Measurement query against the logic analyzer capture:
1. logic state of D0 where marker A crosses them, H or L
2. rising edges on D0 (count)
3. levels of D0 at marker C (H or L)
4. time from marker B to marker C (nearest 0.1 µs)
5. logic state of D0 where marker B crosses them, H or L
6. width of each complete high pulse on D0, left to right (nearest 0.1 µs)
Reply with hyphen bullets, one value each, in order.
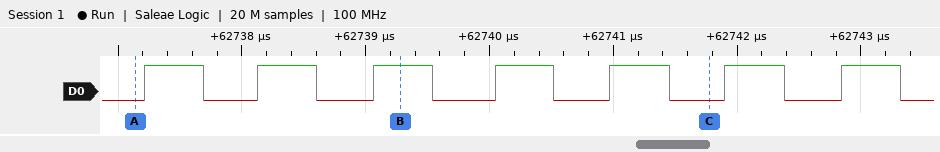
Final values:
- D0=L
- 7
- D0=L
- 2.5 µs
- D0=H
- 0.5 µs, 0.5 µs, 0.5 µs, 0.5 µs, 0.5 µs, 0.5 µs, 0.5 µs
